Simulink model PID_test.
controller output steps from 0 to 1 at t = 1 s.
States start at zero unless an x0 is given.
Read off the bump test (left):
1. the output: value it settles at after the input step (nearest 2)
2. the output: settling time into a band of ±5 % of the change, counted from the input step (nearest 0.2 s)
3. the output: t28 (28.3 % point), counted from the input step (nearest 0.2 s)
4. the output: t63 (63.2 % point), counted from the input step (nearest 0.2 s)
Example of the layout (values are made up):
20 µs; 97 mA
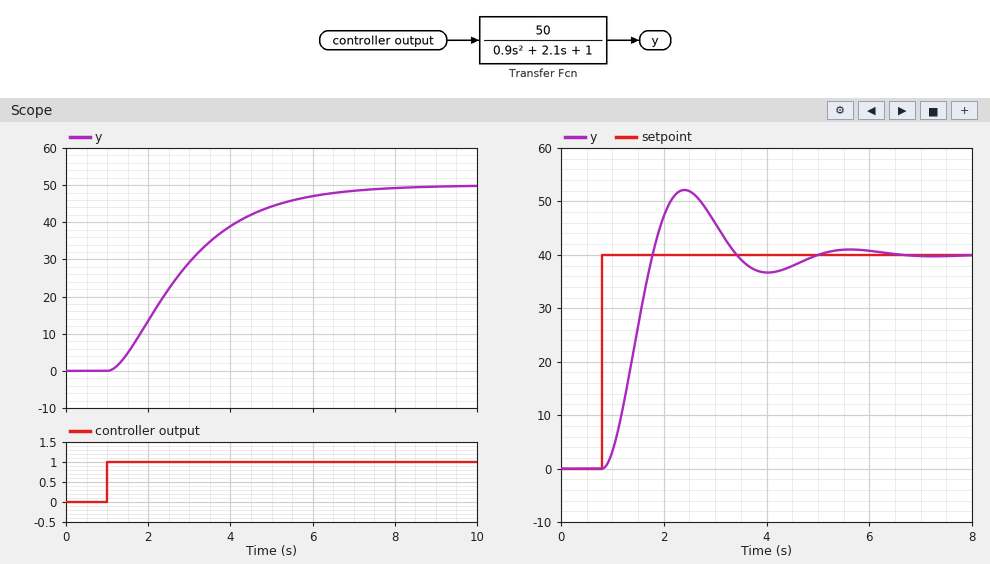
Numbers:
50; 5.2 s; 1.0 s; 2.2 s
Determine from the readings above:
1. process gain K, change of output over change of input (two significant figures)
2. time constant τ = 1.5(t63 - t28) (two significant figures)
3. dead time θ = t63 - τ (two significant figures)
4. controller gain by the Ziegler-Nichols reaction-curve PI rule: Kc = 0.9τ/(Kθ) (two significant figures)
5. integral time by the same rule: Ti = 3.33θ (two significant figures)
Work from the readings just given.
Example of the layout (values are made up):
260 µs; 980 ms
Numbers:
50; 1.8 s; 0.40 s; 0.081; 1.3 s
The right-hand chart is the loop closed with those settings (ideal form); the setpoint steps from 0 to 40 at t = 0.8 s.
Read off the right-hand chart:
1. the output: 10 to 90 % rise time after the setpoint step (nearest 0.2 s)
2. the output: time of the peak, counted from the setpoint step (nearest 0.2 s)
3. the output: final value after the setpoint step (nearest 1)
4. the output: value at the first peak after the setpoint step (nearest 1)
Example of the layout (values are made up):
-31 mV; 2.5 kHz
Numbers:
0.6 s; 1.6 s; 40; 52
